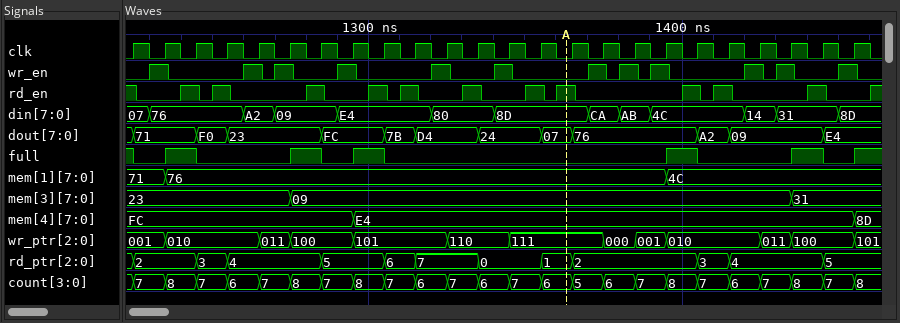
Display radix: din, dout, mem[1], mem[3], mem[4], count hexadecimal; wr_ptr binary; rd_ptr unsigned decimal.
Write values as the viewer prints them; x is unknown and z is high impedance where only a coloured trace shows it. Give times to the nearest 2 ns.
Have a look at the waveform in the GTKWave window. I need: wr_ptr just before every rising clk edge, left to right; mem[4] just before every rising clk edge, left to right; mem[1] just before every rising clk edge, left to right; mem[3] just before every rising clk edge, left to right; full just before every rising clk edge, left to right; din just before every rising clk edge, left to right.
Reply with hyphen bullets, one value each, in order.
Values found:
- 001, 001, 010, 010, 010, 011, 100, 100, 101, 101, 101, 110, 110, 111, 111, 111, 000, 001, 010, 010, 010, 011, 100, 100
- FC, FC, FC, FC, FC, FC, FC, FC, E4, E4, E4, E4, E4, E4, E4, E4, E4, E4, E4, E4, E4, E4, E4, E4
- 71, 71, 76, 76, 76, 76, 76, 76, 76, 76, 76, 76, 76, 76, 76, 76, 76, 76, 4C, 4C, 4C, 4C, 4C, 4C
- 23, 23, 23, 23, 23, 23, 09, 09, 09, 09, 09, 09, 09, 09, 09, 09, 09, 09, 09, 09, 09, 09, 31, 31
- 1 0 1 0 0 0 1 0 1 0 0 0 0 0 0 0 0 0 1 0 0 0 1 0
- 07, 76, 76, 76, A2, 09, 09, E4, E4, E4, 80, 80, 8D, 8D, 8D, CA, AB, 4C, 4C, 4C, 14, 31, 31, 8D
